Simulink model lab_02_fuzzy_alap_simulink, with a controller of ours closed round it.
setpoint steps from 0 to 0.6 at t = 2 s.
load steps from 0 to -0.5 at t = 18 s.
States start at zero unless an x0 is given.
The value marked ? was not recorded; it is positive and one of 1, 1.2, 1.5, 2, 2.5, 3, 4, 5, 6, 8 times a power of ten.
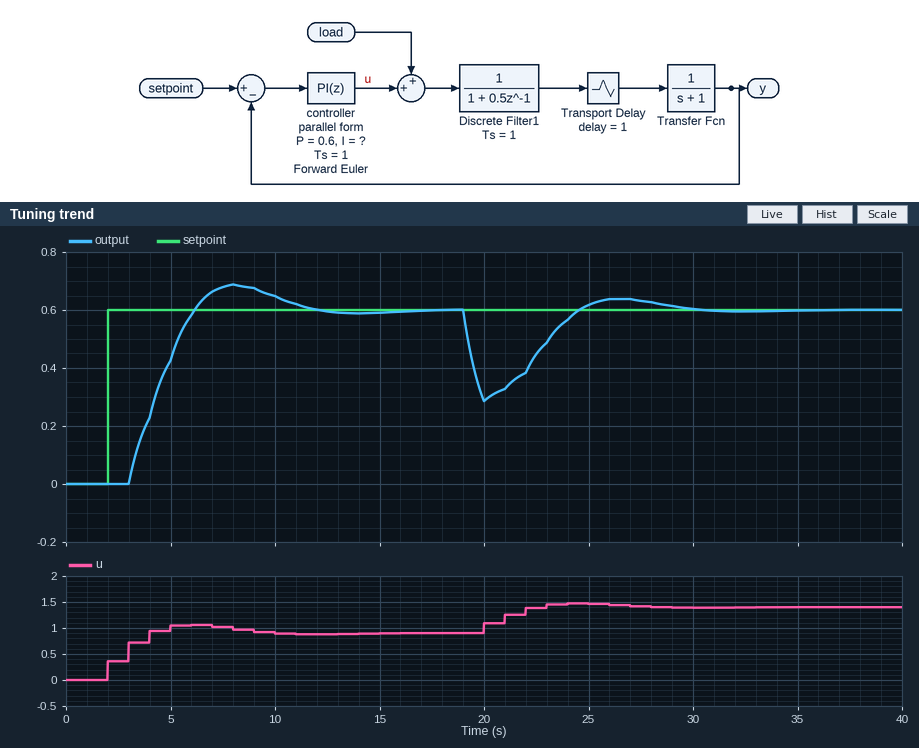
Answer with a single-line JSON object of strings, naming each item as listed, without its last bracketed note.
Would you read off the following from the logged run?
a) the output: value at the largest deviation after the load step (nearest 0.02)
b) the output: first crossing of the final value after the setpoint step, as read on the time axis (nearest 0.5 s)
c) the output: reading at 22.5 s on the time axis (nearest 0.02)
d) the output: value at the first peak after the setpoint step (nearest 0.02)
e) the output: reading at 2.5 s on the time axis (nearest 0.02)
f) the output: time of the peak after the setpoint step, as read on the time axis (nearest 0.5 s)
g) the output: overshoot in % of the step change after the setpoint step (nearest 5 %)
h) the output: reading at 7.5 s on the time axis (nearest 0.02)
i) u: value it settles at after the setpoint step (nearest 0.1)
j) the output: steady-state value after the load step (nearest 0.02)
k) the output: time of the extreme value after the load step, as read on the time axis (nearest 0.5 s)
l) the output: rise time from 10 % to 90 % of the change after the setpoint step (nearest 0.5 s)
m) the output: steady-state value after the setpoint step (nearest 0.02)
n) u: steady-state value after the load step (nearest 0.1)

{"the output: value at the largest deviation after the load step": "0.28", "the output: first crossing of the final value after the setpoint step, as read on the time axis": "6.0 s", "the output: reading at 22.5 s on the time axis": "0.44", "the output: value at the first peak after the setpoint step": "0.68", "the output: reading at 2.5 s on the time axis": "0.00", "the output: time of the peak after the setpoint step, as read on the time axis": "8.0 s", "the output: overshoot in % of the step change after the setpoint step": "15 %", "the output: reading at 7.5 s on the time axis": "0.68", "u: value it settles at after the setpoint step": "0.9", "the output: steady-state value after the load step": "0.60", "the output: time of the extreme value after the load step, as read on the time axis": "20.0 s", "the output: rise time from 10 % to 90 % of the change after the setpoint step": "2.5 s", "the output: steady-state value after the setpoint step": "0.60", "u: steady-state value after the load step": "1.4"}
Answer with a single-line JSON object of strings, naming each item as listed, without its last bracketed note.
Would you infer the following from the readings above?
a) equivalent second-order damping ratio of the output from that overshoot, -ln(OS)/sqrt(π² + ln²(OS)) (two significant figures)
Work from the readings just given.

{"equivalent second-order damping ratio of the output from that overshoot, -ln(OS)/sqrt(π² + ln²(OS))": "0.52"}
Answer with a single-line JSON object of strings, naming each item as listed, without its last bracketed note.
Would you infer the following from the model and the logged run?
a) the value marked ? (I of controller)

{"the value marked ?": "0.6"}
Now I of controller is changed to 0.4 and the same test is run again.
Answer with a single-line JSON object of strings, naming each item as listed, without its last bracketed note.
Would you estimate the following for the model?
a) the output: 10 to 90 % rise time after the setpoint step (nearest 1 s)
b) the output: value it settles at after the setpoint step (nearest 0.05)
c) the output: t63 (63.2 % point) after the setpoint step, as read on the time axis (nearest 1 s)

{"the output: 10 to 90 % rise time after the setpoint step": "5 s", "the output: value it settles at after the setpoint step": "0.60", "the output: t63 (63.2 % point) after the setpoint step, as read on the time axis": "5 s"}
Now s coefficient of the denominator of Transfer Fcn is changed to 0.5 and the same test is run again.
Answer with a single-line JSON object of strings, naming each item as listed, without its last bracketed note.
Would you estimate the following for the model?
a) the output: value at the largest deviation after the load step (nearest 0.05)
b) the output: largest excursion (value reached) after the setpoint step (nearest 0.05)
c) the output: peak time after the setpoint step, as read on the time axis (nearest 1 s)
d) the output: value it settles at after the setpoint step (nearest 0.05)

{"the output: value at the largest deviation after the load step": "0.15", "the output: largest excursion (value reached) after the setpoint step": "0.65", "the output: peak time after the setpoint step, as read on the time axis": "7 s", "the output: value it settles at after the setpoint step": "0.60"}
